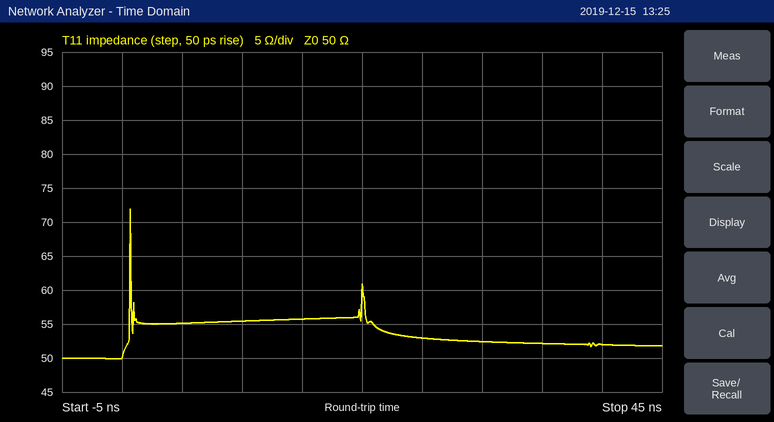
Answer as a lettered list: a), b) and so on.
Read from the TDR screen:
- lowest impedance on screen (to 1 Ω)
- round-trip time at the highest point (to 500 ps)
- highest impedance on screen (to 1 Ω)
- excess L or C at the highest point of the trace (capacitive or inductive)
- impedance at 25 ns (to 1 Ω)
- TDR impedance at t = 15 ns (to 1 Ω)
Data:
a) 50 Ω
b) 500 ps
c) 72 Ω
d) inductive
e) 53 Ω
f) 56 Ω
